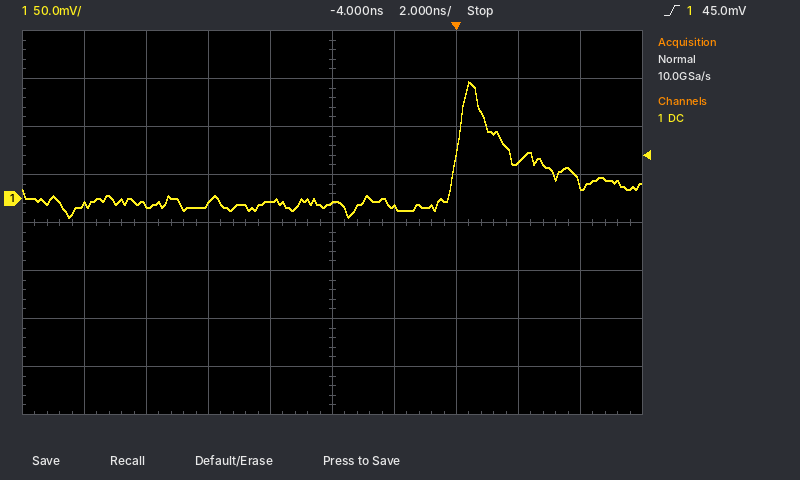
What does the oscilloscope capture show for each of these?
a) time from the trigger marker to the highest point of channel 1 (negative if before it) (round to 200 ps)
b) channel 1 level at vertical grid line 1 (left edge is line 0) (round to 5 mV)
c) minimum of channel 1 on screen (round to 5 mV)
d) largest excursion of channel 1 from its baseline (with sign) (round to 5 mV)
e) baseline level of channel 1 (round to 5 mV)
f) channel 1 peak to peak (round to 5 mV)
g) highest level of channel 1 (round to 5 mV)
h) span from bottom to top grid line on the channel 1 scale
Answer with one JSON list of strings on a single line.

["+400 ps", "-5 mV", "-20 mV", "+125 mV", "-5 mV", "140 mV", "120 mV", "400 mV"]
